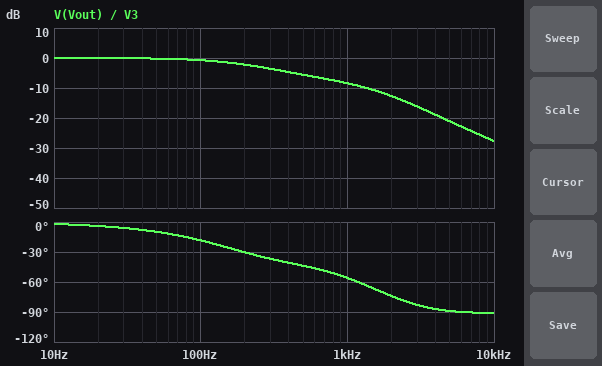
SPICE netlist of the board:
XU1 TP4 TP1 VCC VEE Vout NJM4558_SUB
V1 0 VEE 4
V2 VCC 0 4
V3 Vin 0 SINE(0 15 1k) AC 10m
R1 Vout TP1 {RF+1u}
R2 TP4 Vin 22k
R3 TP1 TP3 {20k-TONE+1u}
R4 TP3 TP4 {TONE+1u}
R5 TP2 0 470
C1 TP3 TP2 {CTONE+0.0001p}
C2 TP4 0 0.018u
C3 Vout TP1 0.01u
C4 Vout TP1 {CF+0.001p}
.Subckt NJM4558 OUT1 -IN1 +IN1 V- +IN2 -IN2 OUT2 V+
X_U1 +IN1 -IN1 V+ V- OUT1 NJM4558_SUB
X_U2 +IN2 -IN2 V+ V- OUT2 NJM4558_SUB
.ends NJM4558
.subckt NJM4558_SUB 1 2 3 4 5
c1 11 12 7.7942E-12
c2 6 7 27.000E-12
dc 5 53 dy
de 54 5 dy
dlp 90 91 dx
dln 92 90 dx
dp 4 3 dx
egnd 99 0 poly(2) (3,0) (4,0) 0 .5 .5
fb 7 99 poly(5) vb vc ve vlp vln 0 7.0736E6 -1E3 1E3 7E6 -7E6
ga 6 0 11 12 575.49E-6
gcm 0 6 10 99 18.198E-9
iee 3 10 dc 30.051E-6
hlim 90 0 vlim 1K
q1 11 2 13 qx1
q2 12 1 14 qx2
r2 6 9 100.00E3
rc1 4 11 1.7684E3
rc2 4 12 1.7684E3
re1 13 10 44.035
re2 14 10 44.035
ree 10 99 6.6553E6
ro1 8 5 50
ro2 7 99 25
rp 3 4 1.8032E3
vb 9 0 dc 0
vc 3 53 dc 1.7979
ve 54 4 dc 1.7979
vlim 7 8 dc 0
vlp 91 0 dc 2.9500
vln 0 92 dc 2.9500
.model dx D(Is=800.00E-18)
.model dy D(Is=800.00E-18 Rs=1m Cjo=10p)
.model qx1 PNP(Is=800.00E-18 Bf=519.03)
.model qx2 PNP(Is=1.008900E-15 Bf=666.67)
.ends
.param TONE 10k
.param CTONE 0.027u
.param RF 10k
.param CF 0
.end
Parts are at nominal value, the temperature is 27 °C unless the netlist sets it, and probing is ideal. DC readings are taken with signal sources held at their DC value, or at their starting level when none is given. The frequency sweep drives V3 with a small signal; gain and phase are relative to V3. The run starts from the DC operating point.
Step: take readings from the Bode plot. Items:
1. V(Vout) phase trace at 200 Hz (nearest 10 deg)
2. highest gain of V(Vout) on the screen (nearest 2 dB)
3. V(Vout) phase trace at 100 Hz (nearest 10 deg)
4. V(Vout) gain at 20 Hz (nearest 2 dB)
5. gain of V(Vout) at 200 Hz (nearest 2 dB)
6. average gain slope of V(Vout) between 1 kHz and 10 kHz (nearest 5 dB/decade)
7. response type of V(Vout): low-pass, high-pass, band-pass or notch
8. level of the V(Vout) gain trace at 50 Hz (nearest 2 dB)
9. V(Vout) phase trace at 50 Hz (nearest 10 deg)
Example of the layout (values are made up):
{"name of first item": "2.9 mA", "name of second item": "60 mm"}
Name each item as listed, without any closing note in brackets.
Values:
{"V(Vout) phase trace at 200 Hz": "-30 deg", "highest gain of V(Vout) on the screen": "0 dB", "V(Vout) phase trace at 100 Hz": "-20 deg", "V(Vout) gain at 20 Hz": "0 dB", "gain of V(Vout) at 200 Hz": "-2 dB", "average gain slope of V(Vout) between 1 kHz and 10 kHz": "-20 dB/decade", "response type of V(Vout): low-pass, high-pass, band-pass or notch": "low-pass", "level of the V(Vout) gain trace at 50 Hz": "0 dB", "V(Vout) phase trace at 50 Hz": "-10 deg"}
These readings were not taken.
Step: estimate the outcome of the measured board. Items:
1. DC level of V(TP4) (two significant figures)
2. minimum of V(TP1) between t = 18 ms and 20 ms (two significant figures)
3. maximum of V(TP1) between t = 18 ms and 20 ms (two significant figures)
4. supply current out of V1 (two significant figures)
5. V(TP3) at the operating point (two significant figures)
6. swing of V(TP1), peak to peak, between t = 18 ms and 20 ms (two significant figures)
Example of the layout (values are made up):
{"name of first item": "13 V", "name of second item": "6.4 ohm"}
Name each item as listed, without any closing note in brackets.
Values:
{"DC level of V(TP4)": "-6.1 mV", "minimum of V(TP1) between t = 18 ms and 20 ms": "-2.5 V", "maximum of V(TP1) between t = 18 ms and 20 ms": "2.5 V", "supply current out of V1": "4.5 mA", "V(TP3) at the operating point": "-9.1 mV", "swing of V(TP1), peak to peak, between t = 18 ms and 20 ms": "5.1 V"}
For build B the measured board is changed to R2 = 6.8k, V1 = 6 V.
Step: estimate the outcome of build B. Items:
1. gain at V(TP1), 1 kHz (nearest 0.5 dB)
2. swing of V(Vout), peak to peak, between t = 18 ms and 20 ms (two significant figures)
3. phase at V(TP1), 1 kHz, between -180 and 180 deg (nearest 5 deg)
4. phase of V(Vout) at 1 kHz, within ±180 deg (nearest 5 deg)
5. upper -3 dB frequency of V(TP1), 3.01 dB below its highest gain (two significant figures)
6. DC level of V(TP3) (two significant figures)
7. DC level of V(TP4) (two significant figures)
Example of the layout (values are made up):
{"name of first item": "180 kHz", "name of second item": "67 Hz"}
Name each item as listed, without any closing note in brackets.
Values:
{"gain at V(TP1), 1 kHz": "-4.5 dB", "swing of V(Vout), peak to peak, between t = 18 ms and 20 ms": "7.9 V", "phase at V(TP1), 1 kHz, between -180 and 180 deg": "-40 deg", "phase of V(Vout) at 1 kHz, within ±180 deg": "-35 deg", "upper -3 dB frequency of V(TP1), 3.01 dB below its highest gain": "670 Hz", "DC level of V(TP3)": "-4.9 mV", "DC level of V(TP4)": "-1.9 mV"}
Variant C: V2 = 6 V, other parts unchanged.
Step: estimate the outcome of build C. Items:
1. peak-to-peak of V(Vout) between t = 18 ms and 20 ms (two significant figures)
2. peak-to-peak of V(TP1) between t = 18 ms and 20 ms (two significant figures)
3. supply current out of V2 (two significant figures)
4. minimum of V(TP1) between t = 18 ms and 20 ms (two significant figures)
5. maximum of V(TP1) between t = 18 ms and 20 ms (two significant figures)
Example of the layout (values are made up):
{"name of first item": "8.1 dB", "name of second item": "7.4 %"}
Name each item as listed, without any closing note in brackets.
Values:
{"peak-to-peak of V(Vout) between t = 18 ms and 20 ms": "7.9 V", "peak-to-peak of V(TP1) between t = 18 ms and 20 ms": "6.1 V", "supply current out of V2": "5.6 mA", "minimum of V(TP1) between t = 18 ms and 20 ms": "-2.4 V", "maximum of V(TP1) between t = 18 ms and 20 ms": "3.7 V"}
